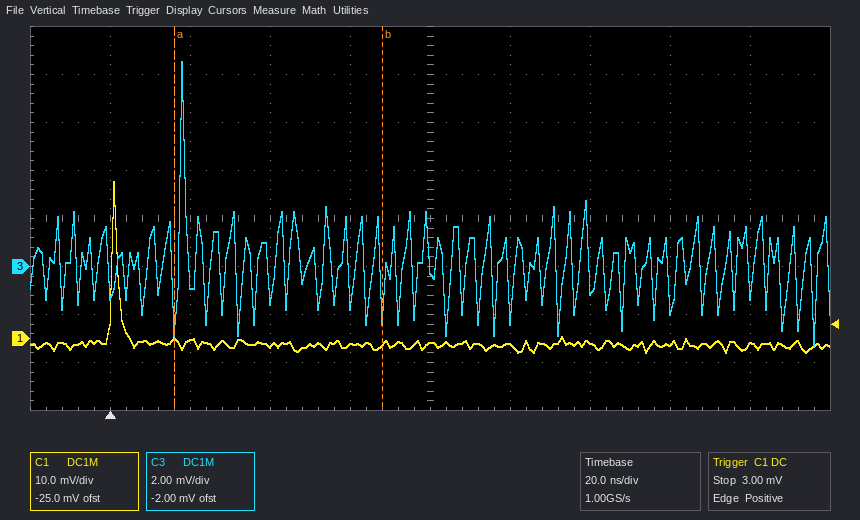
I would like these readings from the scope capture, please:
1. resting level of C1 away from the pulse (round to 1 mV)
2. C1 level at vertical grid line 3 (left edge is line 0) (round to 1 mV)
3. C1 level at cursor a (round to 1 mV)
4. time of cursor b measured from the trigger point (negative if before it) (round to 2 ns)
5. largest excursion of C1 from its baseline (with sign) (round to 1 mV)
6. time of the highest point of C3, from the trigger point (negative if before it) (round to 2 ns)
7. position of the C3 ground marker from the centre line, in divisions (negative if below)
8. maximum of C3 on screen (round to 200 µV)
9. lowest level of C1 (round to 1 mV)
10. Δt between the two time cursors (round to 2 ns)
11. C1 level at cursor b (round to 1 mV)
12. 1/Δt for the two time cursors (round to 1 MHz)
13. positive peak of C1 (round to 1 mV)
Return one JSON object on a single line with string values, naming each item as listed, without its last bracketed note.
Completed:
{"resting level of C1 away from the pulse": "-1 mV", "C1 level at vertical grid line 3 (left edge is line 0)": "-1 mV", "C1 level at cursor a": "0 mV", "time of cursor b measured from the trigger point (negative if before it)": "+68 ns", "largest excursion of C1 from its baseline (with sign)": "+34 mV", "time of the highest point of C3, from the trigger point (negative if before it)": "+18 ns", "position of the C3 ground marker from the centre line, in divisions": "-1.0 div", "maximum of C3 on screen": "8.6 mV", "lowest level of C1": "-3 mV", "Δt between the two time cursors": "52 ns", "C1 level at cursor b": "-1 mV", "1/Δt for the two time cursors": "19 MHz", "positive peak of C1": "33 mV"}
